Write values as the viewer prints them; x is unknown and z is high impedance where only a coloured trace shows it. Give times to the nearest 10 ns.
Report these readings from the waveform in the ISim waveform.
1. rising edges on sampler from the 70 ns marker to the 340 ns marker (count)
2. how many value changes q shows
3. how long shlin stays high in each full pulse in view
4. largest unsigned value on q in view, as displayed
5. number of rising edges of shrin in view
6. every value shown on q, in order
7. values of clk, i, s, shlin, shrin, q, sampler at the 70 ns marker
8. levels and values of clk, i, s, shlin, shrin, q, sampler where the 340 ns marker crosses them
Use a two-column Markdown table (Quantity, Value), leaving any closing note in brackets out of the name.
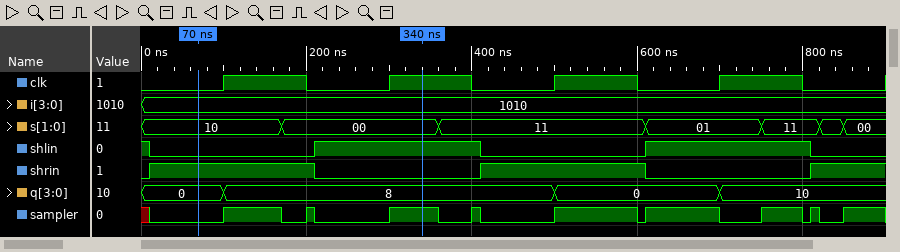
| Quantity | Value |
|---|---|
| rising edges on sampler from the 70 ns marker to the 340 ns marker | 3 |
| how many value changes q shows | 3 |
| how long shlin stays high in each full pulse in view | 200 ns, 200 ns |
| largest unsigned value on q in view, as displayed | 10 |
| number of rising edges of shrin in view | 3 |
| every value shown on q, in order | 0, 8, 0, 10 |
| values of clk, i, s, shlin, shrin, q, sampler at the 70 ns marker | clk=0, i=1010, s=10, shlin=0, shrin=1, q=0, sampler=0 |
| levels and values of clk, i, s, shlin, shrin, q, sampler where the 340 ns marker crosses them | clk=1, i=1010, s=00, shlin=1, shrin=0, q=8, sampler=1 |
